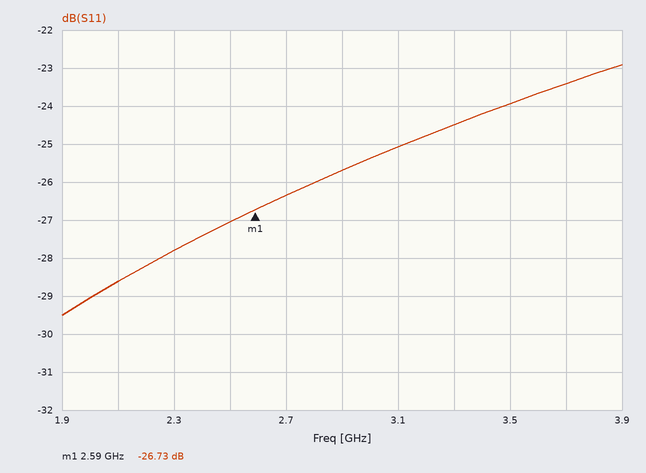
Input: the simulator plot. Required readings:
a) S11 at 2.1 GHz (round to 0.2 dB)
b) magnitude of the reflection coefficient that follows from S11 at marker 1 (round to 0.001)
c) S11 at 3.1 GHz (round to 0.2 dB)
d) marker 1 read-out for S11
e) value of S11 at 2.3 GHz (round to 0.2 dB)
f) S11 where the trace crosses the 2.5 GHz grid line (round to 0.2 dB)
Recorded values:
-28.6 dB
0.046
-25.0 dB
-26.73 dB
-27.8 dB
-27.0 dB
